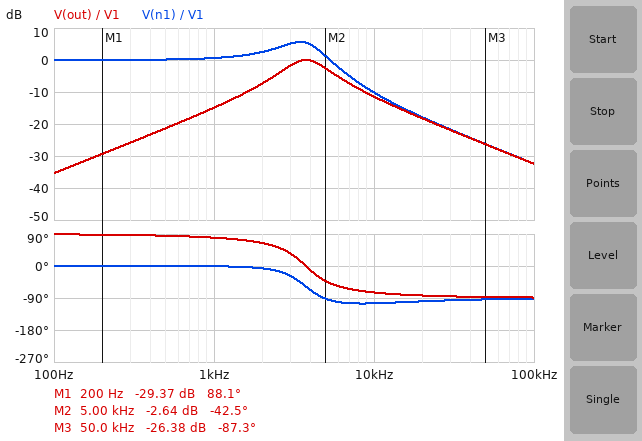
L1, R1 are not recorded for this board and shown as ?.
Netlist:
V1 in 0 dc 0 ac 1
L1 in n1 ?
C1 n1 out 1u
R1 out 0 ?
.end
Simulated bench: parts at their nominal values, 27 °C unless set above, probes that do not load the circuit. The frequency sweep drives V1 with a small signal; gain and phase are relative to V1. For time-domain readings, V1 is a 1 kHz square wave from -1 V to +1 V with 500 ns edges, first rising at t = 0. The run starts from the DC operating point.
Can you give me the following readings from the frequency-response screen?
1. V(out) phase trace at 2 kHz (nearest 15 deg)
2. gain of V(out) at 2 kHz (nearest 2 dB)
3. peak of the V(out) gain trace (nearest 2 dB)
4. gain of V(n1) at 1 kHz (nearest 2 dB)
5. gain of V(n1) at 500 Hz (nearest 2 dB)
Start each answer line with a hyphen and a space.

- 60 deg
- -8 dB
- 0 dB
- 0 dB
- 0 dB
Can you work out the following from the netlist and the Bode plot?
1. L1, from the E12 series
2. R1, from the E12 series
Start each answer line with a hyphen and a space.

- 1.8 mH
- 27 Ω
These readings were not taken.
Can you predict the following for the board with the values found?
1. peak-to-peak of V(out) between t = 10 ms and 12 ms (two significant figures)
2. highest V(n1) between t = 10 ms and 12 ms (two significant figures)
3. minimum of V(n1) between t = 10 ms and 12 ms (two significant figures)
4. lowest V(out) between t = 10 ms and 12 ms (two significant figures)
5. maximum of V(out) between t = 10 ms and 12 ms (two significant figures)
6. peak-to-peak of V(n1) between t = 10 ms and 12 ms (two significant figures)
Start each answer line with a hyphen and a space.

- 1.7 V
- 1.9 V
- -1.9 V
- -840 mV
- 840 mV
- 3.7 V
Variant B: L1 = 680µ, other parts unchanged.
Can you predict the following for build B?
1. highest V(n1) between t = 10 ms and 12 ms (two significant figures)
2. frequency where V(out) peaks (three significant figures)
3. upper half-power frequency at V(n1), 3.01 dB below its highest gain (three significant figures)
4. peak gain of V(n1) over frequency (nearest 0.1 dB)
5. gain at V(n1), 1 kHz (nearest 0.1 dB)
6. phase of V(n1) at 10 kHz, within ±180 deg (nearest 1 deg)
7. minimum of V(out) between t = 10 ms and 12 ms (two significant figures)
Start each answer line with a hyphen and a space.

- 1.6 V
- 6.10 kHz
- 8.49 kHz
- 3.2 dB
- 0.2 dB
- -75 deg
- -1.1 V
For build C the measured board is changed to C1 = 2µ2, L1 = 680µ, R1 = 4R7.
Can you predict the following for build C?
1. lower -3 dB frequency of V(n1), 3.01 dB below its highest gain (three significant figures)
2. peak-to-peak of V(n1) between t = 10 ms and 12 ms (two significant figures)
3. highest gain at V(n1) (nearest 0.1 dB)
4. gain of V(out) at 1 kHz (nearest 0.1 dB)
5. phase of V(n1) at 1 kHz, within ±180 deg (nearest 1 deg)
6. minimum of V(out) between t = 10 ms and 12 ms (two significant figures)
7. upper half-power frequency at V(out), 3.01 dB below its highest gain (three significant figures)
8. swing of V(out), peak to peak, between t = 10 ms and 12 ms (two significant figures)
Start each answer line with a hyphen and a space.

- 3.45 kHz
- 4.3 V
- 11.8 dB
- -23.2 dB
- 0 deg
- -370 mV
- 4.70 kHz
- 750 mV
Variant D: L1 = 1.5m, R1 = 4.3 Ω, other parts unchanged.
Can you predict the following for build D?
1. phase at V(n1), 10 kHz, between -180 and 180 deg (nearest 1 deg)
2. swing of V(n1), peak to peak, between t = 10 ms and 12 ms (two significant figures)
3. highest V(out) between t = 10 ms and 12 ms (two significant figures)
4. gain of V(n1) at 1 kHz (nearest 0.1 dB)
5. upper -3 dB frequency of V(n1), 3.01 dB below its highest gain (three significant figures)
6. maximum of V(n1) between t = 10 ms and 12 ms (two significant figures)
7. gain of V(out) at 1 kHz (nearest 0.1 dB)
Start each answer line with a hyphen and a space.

- -162 deg
- 4.3 V
- 140 mV
- 0.5 dB
- 4.32 kHz
- 2.1 V
- -30.8 dB
